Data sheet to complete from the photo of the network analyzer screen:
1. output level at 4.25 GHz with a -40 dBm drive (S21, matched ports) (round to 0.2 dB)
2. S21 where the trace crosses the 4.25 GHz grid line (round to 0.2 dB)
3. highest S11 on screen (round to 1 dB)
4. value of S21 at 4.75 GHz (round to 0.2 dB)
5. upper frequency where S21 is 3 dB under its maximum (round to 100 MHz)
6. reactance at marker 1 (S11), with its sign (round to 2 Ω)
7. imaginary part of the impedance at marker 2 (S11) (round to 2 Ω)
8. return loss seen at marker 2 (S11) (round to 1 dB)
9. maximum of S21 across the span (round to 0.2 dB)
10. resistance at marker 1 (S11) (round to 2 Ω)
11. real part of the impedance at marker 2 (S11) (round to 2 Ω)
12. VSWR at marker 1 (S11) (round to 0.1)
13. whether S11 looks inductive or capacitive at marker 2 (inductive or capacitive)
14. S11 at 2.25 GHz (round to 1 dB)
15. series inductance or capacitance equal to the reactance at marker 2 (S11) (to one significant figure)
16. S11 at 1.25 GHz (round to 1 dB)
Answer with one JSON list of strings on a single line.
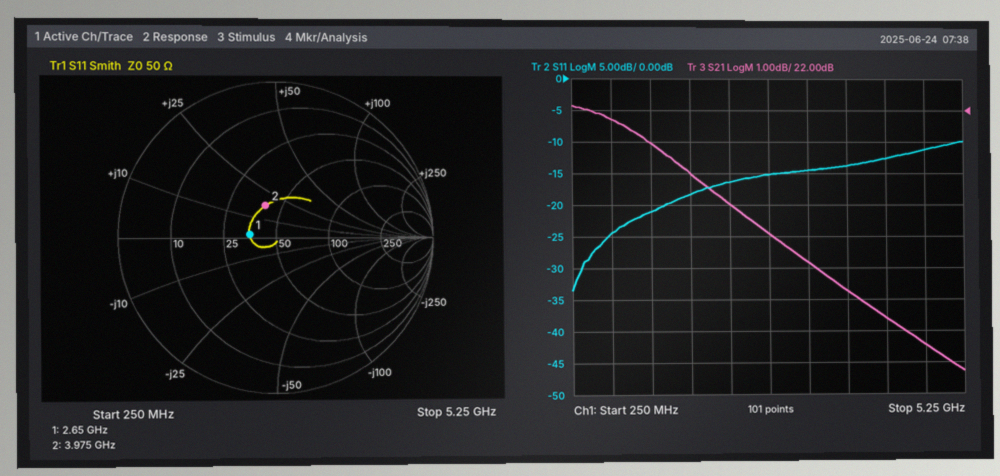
["-24.6 dBm", "15.4 dB", "-10 dB", "14.6 dB", "2.2 GHz", "+2 Ω", "+18 Ω", "13 dB", "22.2 dB", "36 Ω", "40 Ω", "1.4", "inductive", "-16 dB", "700 pH", "-21 dB"]
